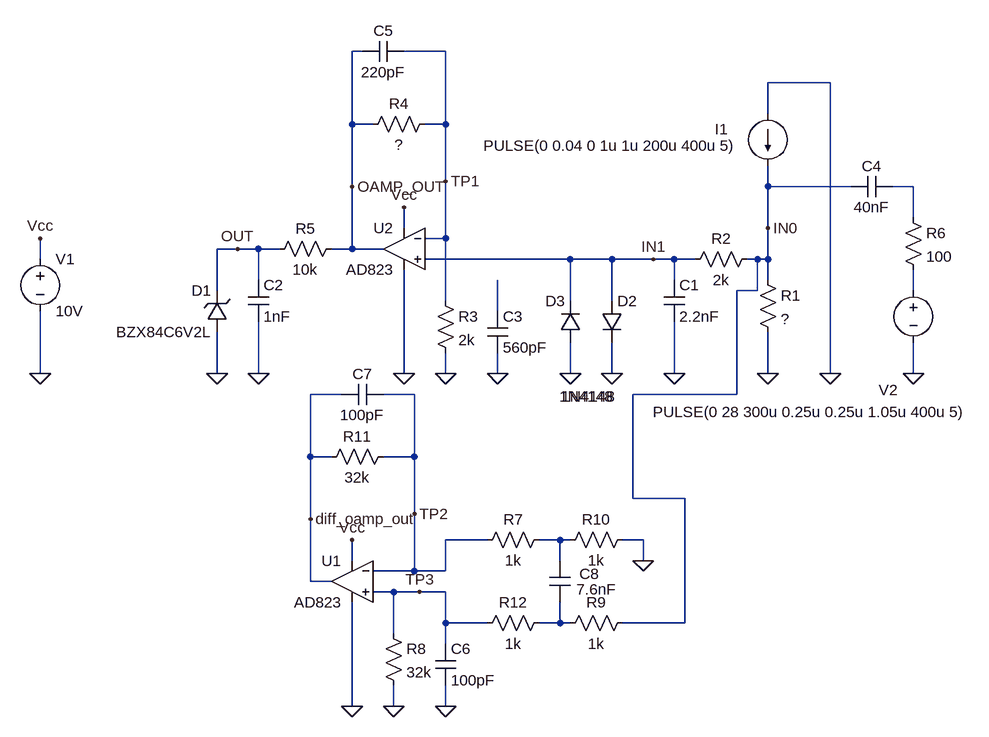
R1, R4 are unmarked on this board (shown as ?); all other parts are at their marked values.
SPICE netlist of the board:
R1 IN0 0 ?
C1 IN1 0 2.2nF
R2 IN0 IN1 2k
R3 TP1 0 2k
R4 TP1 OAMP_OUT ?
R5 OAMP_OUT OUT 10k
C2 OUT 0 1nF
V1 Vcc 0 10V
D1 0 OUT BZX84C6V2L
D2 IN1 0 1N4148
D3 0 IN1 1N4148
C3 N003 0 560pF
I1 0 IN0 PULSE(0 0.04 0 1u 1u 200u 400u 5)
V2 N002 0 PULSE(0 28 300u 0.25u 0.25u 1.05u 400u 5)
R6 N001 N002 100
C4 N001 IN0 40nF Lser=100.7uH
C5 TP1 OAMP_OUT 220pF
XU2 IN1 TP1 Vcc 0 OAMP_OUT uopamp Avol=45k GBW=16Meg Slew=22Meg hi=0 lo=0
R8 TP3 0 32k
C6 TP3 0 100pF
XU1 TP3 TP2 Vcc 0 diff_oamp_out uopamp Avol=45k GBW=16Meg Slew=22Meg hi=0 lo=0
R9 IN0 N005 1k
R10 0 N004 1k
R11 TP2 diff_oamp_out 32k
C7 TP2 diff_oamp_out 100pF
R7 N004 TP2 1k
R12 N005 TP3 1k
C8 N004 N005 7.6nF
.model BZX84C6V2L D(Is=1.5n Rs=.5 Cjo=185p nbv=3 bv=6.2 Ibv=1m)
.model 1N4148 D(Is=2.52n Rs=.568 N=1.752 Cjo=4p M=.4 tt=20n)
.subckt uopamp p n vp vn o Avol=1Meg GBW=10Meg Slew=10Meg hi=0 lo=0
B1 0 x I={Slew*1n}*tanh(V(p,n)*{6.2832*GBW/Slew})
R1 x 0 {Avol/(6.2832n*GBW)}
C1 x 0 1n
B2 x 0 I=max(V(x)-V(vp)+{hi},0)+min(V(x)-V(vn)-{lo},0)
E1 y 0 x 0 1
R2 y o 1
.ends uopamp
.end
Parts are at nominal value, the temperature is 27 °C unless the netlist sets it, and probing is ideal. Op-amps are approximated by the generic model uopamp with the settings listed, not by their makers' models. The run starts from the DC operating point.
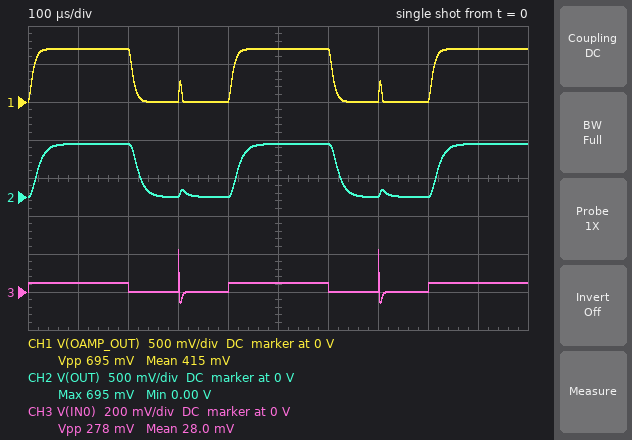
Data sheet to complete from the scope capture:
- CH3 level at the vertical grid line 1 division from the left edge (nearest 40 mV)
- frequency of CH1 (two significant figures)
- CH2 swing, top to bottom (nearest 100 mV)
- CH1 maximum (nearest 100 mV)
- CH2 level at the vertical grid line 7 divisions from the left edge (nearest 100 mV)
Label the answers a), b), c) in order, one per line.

a) 40 mV
b) 2.5 kHz
c) 700 mV
d) 700 mV
e) 0 V
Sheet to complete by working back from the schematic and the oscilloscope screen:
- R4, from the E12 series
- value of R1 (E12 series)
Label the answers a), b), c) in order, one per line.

a) 27 kΩ
b) 1.2 Ω
